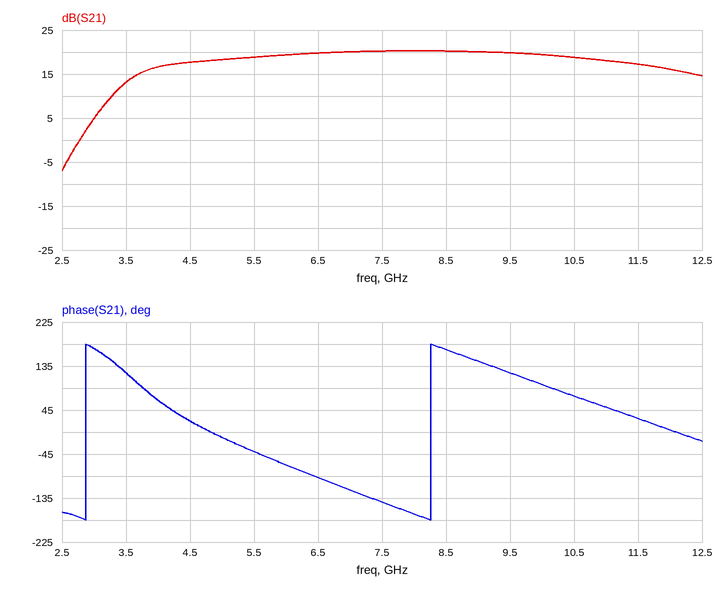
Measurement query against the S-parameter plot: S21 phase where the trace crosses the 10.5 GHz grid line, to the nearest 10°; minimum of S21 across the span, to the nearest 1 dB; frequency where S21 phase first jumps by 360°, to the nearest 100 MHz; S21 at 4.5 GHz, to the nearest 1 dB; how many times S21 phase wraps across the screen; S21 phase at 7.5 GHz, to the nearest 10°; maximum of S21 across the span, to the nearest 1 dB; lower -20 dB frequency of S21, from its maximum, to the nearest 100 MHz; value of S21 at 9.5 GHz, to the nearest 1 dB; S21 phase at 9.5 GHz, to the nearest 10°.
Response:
70°
-7 dB
2.9 GHz
18 dB
2
-140°
20 dB
2.8 GHz
20 dB
120°
